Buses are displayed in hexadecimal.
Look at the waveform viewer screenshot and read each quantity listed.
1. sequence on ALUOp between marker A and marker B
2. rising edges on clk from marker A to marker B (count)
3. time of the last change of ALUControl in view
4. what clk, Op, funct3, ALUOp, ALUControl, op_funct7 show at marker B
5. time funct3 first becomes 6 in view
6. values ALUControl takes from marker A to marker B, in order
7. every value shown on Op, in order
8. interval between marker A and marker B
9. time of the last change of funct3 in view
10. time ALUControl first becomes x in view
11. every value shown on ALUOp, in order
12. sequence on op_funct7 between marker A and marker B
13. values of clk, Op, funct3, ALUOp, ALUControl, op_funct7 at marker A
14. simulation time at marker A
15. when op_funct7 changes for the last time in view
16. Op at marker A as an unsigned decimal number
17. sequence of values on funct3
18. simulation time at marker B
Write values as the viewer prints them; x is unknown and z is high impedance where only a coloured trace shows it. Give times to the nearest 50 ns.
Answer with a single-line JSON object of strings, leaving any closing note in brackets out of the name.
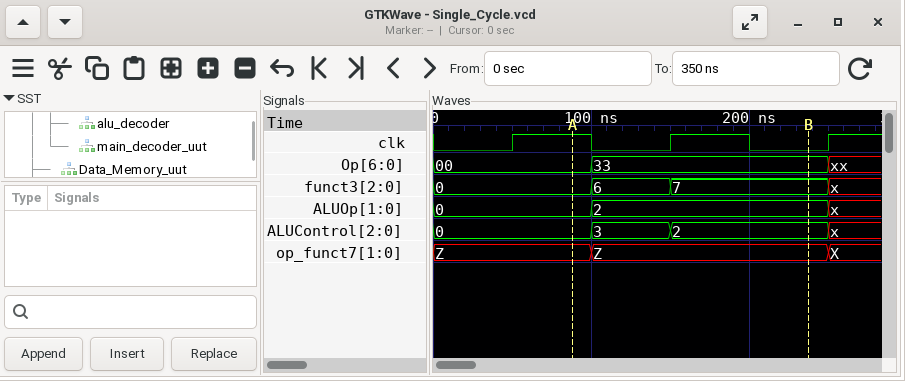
{"sequence on ALUOp between marker A and marker B": "0, 2", "rising edges on clk from marker A to marker B": "1", "time of the last change of ALUControl in view": "250 ns", "what clk, Op, funct3, ALUOp, ALUControl, op_funct7 show at marker B": "clk=0, Op=33, funct3=7, ALUOp=2, ALUControl=2, op_funct7=Z", "time funct3 first becomes 6 in view": "100 ns", "values ALUControl takes from marker A to marker B, in order": "0, 3, 2", "every value shown on Op, in order": "00, 33, xx", "interval between marker A and marker B": "150 ns", "time of the last change of funct3 in view": "250 ns", "time ALUControl first becomes x in view": "250 ns", "every value shown on ALUOp, in order": "0, 2, x", "sequence on op_funct7 between marker A and marker B": "Z, Z", "values of clk, Op, funct3, ALUOp, ALUControl, op_funct7 at marker A": "clk=1, Op=00, funct3=0, ALUOp=0, ALUControl=0, op_funct7=Z", "simulation time at marker A": "100 ns", "when op_funct7 changes for the last time in view": "250 ns", "Op at marker A as an unsigned decimal number": "0", "sequence of values on funct3": "0, 6, 7, x", "simulation time at marker B": "250 ns"}
